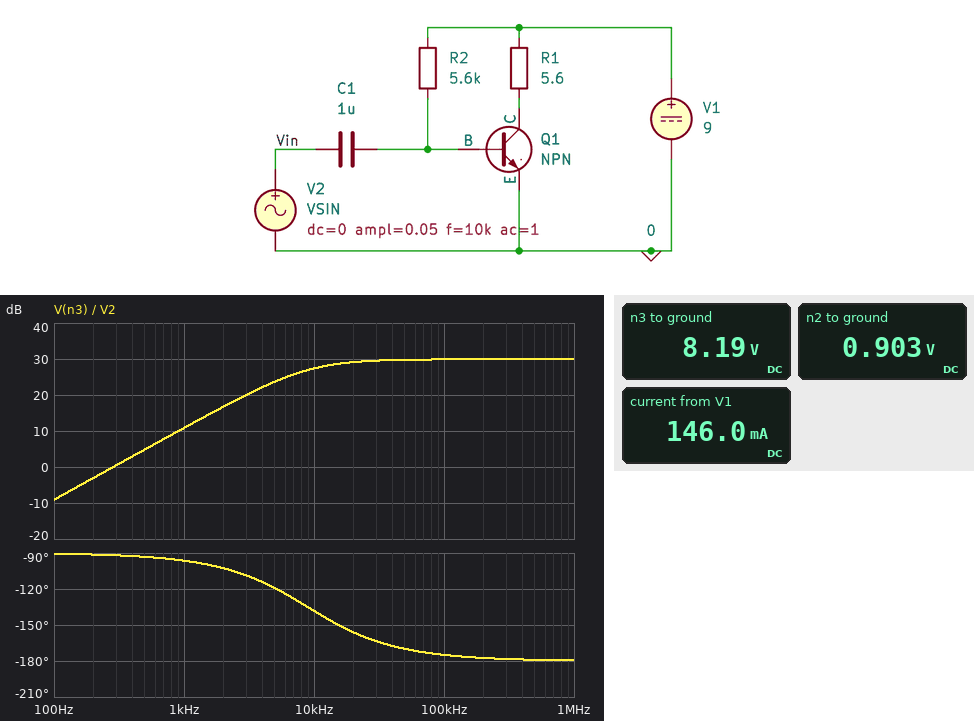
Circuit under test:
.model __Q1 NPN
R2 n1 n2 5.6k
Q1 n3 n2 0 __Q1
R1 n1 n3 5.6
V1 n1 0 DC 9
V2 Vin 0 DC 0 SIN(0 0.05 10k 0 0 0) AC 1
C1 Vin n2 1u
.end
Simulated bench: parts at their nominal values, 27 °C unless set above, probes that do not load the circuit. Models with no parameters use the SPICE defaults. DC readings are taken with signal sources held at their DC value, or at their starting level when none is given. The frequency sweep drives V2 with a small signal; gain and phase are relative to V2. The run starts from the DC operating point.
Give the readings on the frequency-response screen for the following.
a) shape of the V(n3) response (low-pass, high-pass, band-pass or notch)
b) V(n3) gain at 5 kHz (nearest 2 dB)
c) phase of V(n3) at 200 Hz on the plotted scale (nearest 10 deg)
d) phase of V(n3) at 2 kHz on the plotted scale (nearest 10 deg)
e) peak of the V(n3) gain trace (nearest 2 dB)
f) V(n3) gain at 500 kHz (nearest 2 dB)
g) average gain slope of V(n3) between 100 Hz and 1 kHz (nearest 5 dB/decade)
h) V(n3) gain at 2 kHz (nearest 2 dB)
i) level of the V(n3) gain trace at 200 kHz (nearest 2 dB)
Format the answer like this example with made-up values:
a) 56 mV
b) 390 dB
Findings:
a) high-pass
b) 24 dB
c) -90 deg
d) -100 deg
e) 30 dB
f) 30 dB
g) 20 dB/decade
h) 16 dB
i) 30 dB
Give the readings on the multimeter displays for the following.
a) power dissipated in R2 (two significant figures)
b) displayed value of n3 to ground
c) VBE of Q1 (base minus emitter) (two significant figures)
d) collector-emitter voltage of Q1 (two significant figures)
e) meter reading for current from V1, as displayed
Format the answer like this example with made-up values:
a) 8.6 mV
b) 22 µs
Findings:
a) 12 mW
b) 8.19 V
c) 900 mV
d) 8.2 V
e) 146.0 mA
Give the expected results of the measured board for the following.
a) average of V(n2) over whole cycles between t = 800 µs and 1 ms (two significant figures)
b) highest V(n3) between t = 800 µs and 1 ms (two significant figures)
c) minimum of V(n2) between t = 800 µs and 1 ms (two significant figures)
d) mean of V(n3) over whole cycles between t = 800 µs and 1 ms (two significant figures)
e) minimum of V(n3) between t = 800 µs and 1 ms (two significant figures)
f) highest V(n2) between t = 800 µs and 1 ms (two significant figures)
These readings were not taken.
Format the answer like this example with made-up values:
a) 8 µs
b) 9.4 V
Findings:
a) 890 mV
b) 8.9 V
c) 850 mV
d) 8.2 V
e) 6.9 V
f) 930 mV
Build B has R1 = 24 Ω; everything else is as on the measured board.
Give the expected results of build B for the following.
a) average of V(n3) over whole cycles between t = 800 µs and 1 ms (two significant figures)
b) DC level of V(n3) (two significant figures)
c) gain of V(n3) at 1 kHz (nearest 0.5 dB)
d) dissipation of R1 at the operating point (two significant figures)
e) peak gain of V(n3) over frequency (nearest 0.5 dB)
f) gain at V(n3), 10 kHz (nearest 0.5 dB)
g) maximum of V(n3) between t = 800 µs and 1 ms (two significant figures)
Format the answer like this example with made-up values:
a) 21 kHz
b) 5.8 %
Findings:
a) 5.6 V
b) 5.5 V
c) 23.5 dB
d) 500 mW
e) 42.5 dB
f) 40.0 dB
g) 8.6 V
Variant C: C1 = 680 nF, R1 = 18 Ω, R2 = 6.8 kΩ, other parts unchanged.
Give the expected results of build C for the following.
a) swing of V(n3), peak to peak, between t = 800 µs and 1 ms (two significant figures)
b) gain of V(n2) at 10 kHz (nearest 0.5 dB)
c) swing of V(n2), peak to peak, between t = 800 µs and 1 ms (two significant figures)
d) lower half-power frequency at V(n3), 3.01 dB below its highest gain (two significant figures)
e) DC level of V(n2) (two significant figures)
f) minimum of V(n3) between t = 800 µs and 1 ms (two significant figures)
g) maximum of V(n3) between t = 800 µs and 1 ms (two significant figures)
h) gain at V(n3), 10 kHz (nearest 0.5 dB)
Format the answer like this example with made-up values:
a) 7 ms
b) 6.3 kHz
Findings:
a) 5.0 V
b) -3.5 dB
c) 74 mV
d) 11 kHz
e) 900 mV
f) 3.7 V
g) 8.7 V
h) 35.0 dB
